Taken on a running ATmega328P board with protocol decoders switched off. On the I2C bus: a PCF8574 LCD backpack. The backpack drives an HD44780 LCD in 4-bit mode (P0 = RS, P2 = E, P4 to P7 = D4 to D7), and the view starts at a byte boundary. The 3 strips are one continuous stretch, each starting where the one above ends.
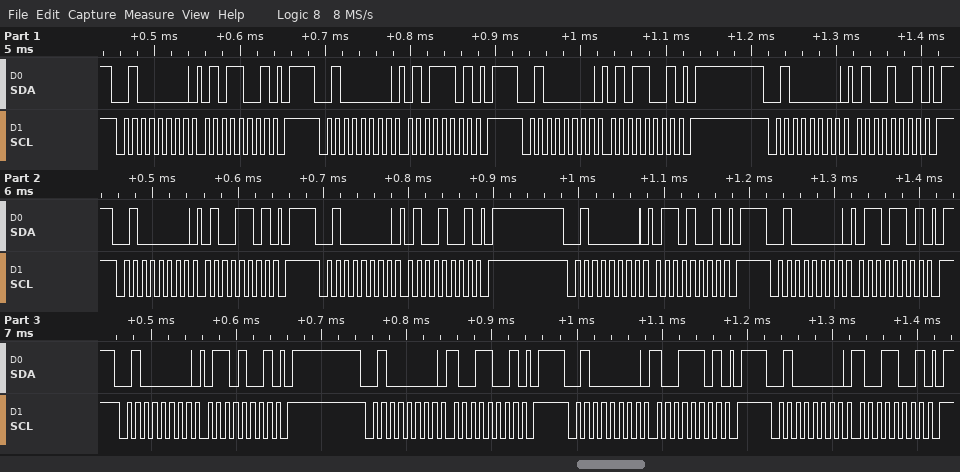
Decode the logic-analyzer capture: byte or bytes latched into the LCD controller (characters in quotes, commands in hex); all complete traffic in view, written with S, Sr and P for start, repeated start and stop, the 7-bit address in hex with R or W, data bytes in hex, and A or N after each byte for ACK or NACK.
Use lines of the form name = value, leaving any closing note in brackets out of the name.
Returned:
byte or bytes latched into the LCD controller = 'T' 'i'
all complete traffic in view, written with S, Sr and P for start, repeated start and stop, the 7-bit address in hex with R or W, data bytes in hex, and A or N after each byte for ACK or NACK = S 20W A 59 A P S 20W A 5D A P S 20W A 59 A P S 20W A 49 A P S 20W A 4D A P S 20W A 49 A P S 20W A 69 A P S 20W A 6D A P S 20W A 69 A P S 20W A 99 A P S 20W A 9D A P S 20W A 99 A P
